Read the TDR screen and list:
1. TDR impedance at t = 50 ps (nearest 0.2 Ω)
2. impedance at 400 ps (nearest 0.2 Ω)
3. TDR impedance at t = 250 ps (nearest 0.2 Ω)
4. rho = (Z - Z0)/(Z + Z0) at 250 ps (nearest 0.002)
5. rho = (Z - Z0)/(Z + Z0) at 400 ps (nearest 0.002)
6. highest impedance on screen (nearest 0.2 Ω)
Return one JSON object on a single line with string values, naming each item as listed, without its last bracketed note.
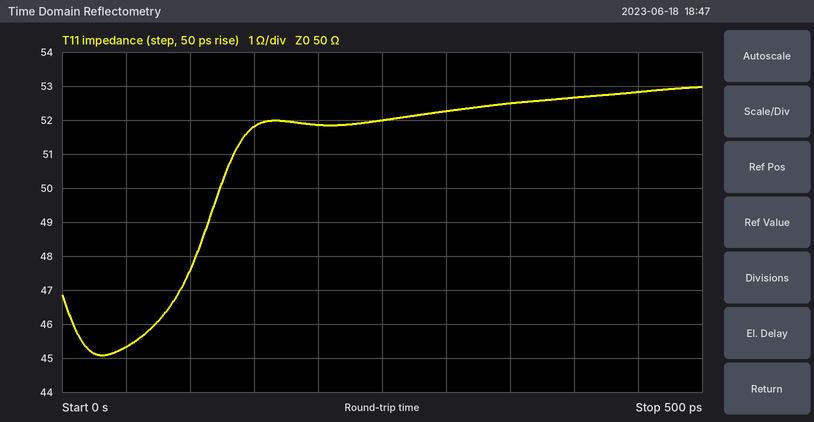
{"TDR impedance at t = 50 ps": "45.4 Ω", "impedance at 400 ps": "52.6 Ω", "TDR impedance at t = 250 ps": "52.0 Ω", "rho = (Z - Z0)/(Z + Z0) at 250 ps": "+0.020", "rho = (Z - Z0)/(Z + Z0) at 400 ps": "+0.026", "highest impedance on screen": "53.0 Ω"}
